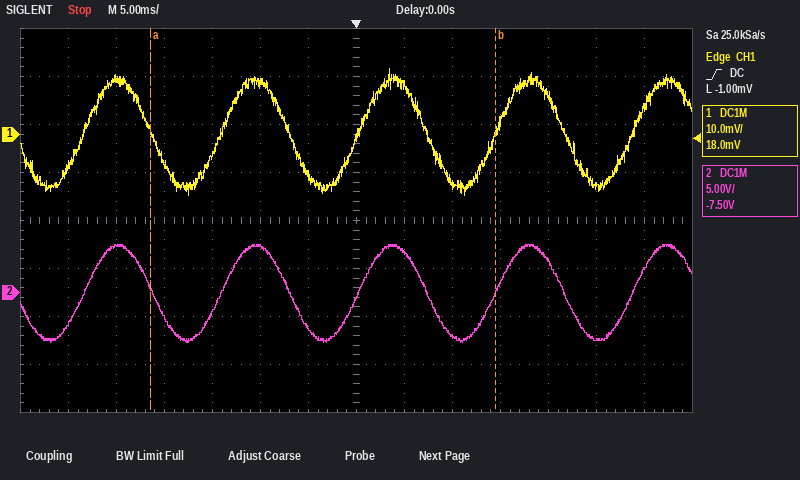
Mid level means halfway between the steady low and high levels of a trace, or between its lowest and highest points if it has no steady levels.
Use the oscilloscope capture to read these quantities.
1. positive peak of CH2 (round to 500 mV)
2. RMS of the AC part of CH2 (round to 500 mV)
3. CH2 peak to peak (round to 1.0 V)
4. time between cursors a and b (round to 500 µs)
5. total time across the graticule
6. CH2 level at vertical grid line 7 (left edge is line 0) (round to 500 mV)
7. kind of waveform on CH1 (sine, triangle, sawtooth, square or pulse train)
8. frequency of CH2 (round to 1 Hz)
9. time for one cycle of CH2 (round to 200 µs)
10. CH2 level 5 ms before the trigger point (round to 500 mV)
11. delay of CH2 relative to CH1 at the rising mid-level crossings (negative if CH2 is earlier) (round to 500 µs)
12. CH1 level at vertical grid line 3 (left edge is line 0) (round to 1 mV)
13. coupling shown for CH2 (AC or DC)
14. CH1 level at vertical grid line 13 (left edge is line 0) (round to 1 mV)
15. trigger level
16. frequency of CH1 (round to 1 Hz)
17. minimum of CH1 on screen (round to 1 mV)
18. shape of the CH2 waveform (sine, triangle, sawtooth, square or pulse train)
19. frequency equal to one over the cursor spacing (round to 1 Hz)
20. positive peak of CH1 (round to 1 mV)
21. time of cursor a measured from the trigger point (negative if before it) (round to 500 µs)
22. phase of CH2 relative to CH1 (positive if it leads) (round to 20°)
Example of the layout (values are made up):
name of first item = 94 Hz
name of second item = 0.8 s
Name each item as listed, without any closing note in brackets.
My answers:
positive peak of CH2 = 5.0 V
RMS of the AC part of CH2 = 3.5 V
CH2 peak to peak = 10.0 V
time between cursors a and b = 36.0 ms
total time across the graticule = 70 ms
CH2 level at vertical grid line 7 (left edge is line 0) = -500 mV
kind of waveform on CH1 = sine
frequency of CH2 = 70 Hz
time for one cycle of CH2 = 14.2 ms
CH2 level 5 ms before the trigger point = -3.5 V
delay of CH2 relative to CH1 at the rising mid-level crossings (negative if CH2 is earlier) = 0.0 ms
CH1 level at vertical grid line 3 (left edge is line 0) = -6 mV
coupling shown for CH2 = DC
CH1 level at vertical grid line 13 (left edge is line 0) = 5 mV
trigger level = -1.00 mV
frequency of CH1 = 70 Hz
minimum of CH1 on screen = -13 mV
shape of the CH2 waveform = sine
frequency equal to one over the cursor spacing = 28 Hz
positive peak of CH1 = 14 mV
time of cursor a measured from the trigger point (negative if before it) = -21.5 ms
phase of CH2 relative to CH1 (positive if it leads) = 0°
